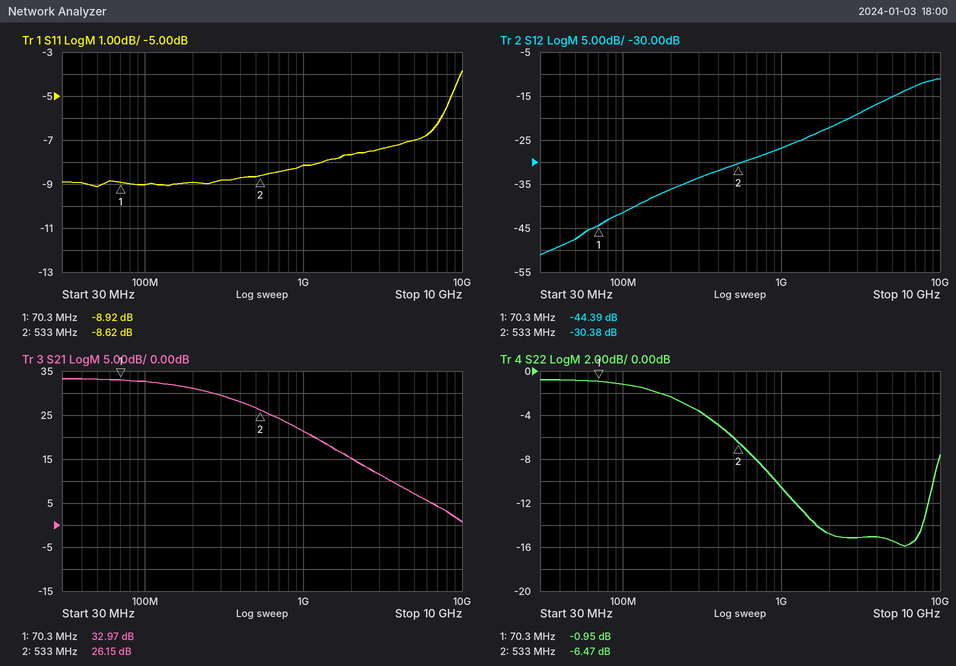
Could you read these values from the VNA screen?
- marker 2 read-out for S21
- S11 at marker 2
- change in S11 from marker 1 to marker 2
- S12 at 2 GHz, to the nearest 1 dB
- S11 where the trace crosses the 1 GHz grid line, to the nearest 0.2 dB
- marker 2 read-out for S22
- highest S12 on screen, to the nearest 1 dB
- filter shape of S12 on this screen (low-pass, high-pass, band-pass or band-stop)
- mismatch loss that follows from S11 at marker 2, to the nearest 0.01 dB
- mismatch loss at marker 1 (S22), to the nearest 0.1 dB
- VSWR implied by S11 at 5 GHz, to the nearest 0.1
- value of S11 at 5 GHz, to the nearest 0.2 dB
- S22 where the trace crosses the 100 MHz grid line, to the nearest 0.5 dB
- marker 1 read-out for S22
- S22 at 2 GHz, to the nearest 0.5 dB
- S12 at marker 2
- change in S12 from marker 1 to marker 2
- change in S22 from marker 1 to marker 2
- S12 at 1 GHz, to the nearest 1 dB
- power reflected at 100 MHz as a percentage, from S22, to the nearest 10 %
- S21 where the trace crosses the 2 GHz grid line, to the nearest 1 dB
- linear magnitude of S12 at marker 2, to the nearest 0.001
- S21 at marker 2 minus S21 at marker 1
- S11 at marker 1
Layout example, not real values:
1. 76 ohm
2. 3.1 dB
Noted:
1. 26.15 dB
2. -8.62 dB
3. 0.30 dB
4. -22 dB
5. -8.2 dB
6. -6.47 dB
7. -11 dB
8. high-pass
9. 0.64 dB
10. 7.1 dB
11. 2.6
12. -7.0 dB
13. -1.0 dB
14. -0.95 dB
15. -15.0 dB
16. -30.38 dB
17. 14.01 dB
18. -5.52 dB
19. -27 dB
20. 80 %
21. 15 dB
22. 0.030
23. -6.82 dB
24. -8.92 dB
